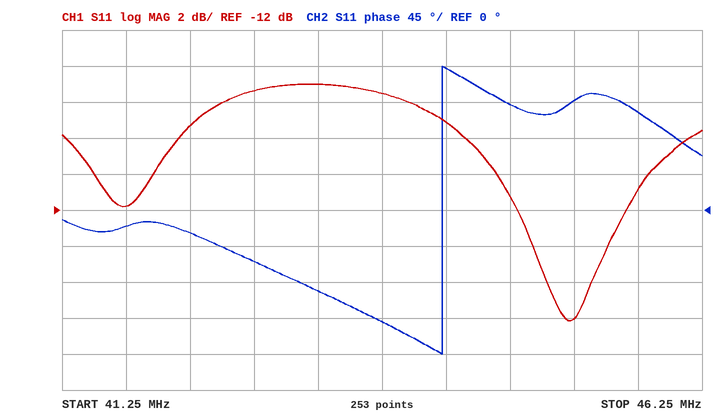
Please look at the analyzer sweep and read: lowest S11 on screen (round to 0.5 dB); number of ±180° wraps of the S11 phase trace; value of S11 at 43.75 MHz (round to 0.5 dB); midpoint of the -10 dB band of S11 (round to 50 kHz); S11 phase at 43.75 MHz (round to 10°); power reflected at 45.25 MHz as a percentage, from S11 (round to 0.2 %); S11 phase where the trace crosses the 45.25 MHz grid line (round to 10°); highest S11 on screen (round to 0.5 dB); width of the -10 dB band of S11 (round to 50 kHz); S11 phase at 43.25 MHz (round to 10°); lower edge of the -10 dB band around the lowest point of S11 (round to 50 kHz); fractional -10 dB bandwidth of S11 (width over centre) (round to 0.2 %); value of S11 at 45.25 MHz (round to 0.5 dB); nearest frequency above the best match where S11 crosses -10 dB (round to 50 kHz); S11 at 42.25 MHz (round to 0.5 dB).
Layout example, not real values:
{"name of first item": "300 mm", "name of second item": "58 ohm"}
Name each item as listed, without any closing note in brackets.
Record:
{"lowest S11 on screen": "-18.0 dB", "number of ±180° wraps of the S11 phase trace": "1", "value of S11 at 43.75 MHz": "-5.5 dB", "midpoint of the -10 dB band of S11": "45.25 MHz", "S11 phase at 43.75 MHz": "-140°", "power reflected at 45.25 MHz as a percentage, from S11": "1.6 %", "S11 phase where the trace crosses the 45.25 MHz grid line": "140°", "highest S11 on screen": "-5.0 dB", "width of the -10 dB band of S11": "1.20 MHz", "S11 phase at 43.25 MHz": "-100°", "lower edge of the -10 dB band around the lowest point of S11": "44.65 MHz", "fractional -10 dB bandwidth of S11 (width over centre)": "2.6 %", "value of S11 at 45.25 MHz": "-18.0 dB", "nearest frequency above the best match where S11 crosses -10 dB": "45.85 MHz", "S11 at 42.25 MHz": "-7.5 dB"}
